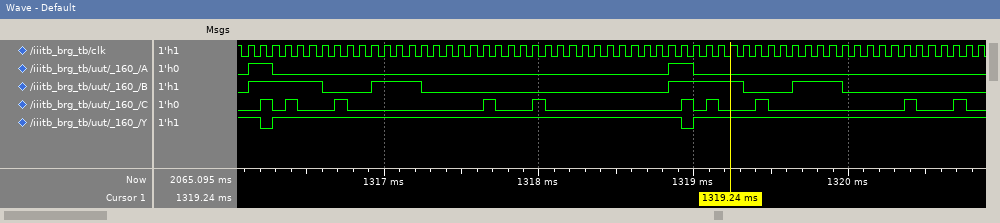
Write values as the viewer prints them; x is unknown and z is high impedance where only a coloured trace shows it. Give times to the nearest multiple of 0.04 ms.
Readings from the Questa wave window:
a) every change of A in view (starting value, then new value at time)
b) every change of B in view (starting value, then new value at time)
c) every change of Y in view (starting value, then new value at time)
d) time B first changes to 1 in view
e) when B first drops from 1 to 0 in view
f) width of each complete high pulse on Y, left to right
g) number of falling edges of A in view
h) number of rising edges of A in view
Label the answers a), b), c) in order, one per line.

a) 0, 1 at 1316.12 ms, 0 at 1316.28 ms, 1 at 1318.84 ms, 0 at 1319 ms
b) 0, 1 at 1316.12 ms, 0 at 1316.6 ms, 1 at 1316.92 ms, 0 at 1317.24 ms, 1 at 1318.84 ms, 0 at 1319.32 ms, 1 at 1319.64 ms, 0 at 1319.96 ms
c) 1, 0 at 1316.2 ms, 1 at 1316.28 ms, 0 at 1318.92 ms, 1 at 1319 ms
d) 1316.12 ms
e) 1316.6 ms
f) 2.64 ms
g) 2
h) 2
